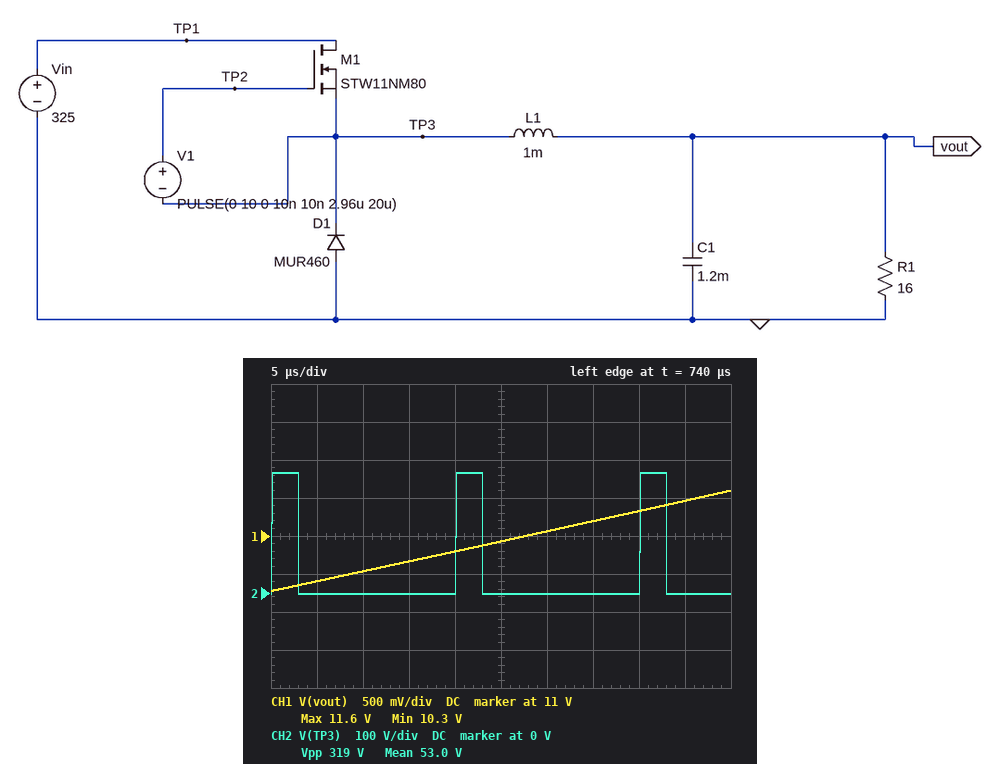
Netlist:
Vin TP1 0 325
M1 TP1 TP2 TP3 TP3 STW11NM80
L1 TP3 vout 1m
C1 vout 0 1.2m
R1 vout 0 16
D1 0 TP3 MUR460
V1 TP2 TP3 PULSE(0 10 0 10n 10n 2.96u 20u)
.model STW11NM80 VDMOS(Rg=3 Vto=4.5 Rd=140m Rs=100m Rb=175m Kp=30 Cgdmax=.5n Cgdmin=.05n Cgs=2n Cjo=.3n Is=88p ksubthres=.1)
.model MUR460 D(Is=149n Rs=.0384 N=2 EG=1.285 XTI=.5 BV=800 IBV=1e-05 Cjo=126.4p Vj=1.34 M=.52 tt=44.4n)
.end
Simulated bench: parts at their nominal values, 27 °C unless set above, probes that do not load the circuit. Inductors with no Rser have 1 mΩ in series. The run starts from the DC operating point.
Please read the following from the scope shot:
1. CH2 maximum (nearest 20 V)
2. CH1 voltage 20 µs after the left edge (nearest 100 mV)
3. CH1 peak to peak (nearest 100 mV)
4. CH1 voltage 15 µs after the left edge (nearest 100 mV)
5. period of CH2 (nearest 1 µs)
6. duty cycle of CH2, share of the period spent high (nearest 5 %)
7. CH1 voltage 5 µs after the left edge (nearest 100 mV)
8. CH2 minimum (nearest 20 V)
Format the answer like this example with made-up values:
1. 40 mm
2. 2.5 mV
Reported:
1. 320 V
2. 10.8 V
3. 1.3 V
4. 10.7 V
5. 20 µs
6. 15 %
7. 10.4 V
8. 0 V
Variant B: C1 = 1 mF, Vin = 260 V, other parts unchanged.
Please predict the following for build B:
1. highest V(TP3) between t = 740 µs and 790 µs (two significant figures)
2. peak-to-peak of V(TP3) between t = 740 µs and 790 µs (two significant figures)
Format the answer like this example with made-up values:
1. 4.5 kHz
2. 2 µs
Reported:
1. 250 V
2. 260 V
